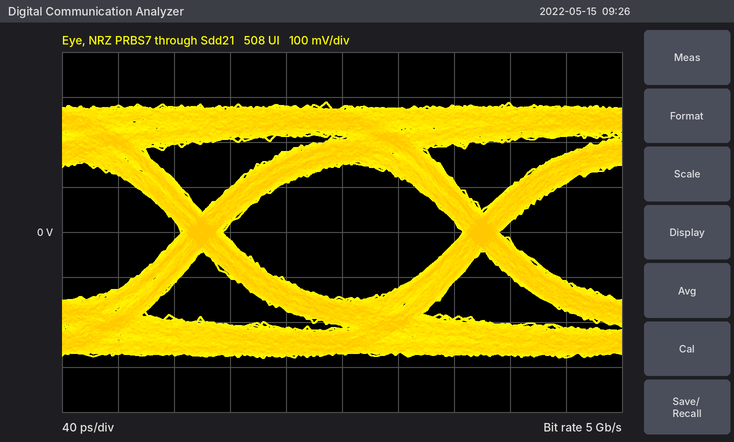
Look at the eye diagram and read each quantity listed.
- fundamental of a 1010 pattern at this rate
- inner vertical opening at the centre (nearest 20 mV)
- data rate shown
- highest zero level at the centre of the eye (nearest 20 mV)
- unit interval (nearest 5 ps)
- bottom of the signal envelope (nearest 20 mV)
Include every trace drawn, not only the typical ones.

2.5 GHz
300 mV
5 Gb/s
-140 mV
200 ps
-280 mV
